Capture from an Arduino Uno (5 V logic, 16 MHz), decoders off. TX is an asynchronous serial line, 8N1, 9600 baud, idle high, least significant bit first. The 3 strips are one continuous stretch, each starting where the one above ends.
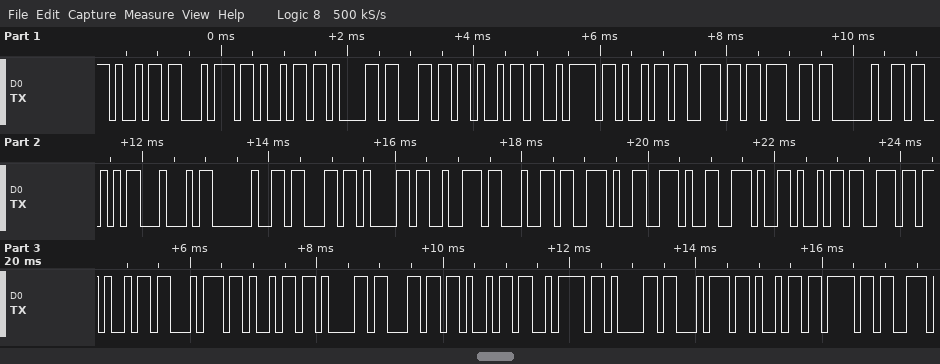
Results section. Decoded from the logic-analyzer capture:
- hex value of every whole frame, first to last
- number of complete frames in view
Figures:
0x69 0x74 0x69 0x61 0x6C 0x69 0x7A 0x69 0x6E 0x67 0x20 0x53 0x44 0x20 0x63 0x61 0x72 0x64 0x2E 0x2E 0x2E 0x69 0x6E 0x69 0x74 0x69 0x61 0x6C 0x69 0x7A 0x61 0x74 0x69 0x6F
34
